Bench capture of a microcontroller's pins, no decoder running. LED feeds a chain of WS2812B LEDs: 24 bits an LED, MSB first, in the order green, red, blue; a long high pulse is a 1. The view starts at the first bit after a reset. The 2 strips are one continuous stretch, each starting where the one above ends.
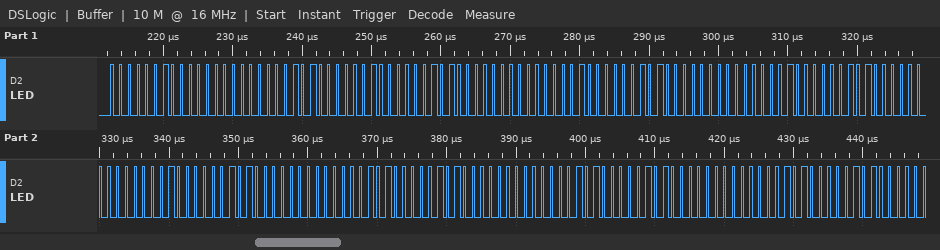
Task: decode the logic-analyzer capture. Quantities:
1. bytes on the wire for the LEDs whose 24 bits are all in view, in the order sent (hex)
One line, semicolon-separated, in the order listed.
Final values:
02 00 05 02 05 00 02 05 00 02 05 00 02 05 00 05 05 00 05 05 00
